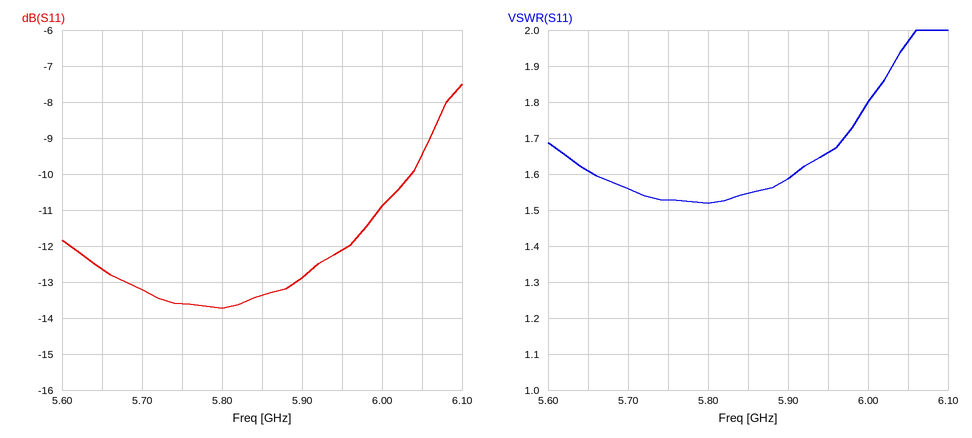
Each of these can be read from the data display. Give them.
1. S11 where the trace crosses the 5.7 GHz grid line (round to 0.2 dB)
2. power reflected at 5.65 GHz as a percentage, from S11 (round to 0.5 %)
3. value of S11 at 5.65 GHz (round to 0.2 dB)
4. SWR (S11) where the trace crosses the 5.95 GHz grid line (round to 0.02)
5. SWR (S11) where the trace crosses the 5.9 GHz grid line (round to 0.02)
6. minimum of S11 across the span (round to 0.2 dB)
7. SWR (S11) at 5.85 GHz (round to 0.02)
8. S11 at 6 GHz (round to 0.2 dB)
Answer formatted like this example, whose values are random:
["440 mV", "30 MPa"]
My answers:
["-13.2 dB", "5.5 %", "-12.6 dB", "1.66", "1.58", "-13.8 dB", "1.54", "-10.8 dB"]
